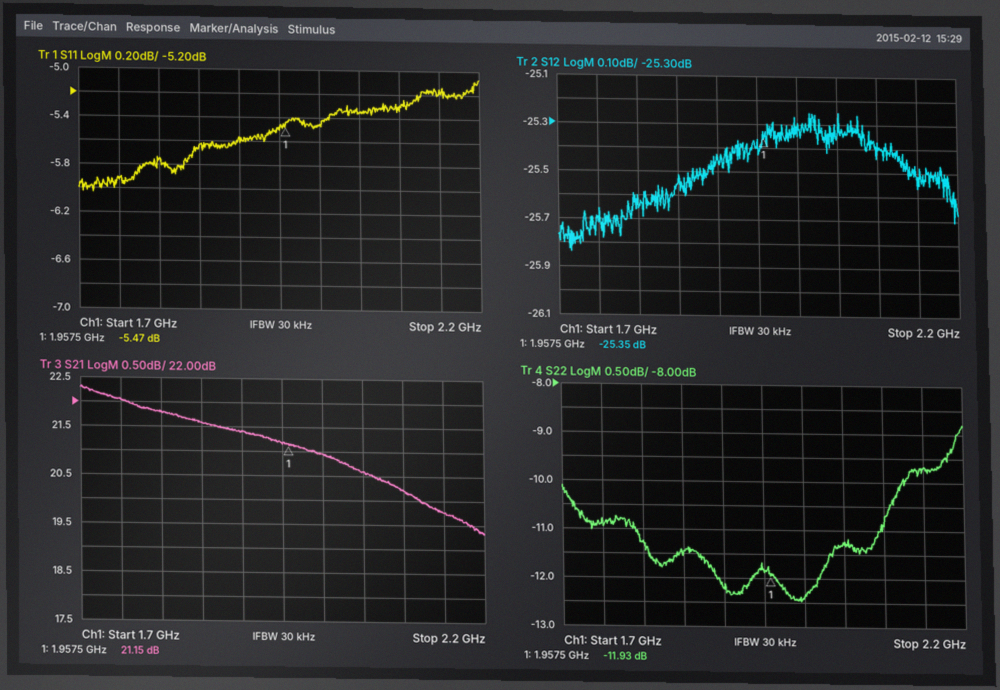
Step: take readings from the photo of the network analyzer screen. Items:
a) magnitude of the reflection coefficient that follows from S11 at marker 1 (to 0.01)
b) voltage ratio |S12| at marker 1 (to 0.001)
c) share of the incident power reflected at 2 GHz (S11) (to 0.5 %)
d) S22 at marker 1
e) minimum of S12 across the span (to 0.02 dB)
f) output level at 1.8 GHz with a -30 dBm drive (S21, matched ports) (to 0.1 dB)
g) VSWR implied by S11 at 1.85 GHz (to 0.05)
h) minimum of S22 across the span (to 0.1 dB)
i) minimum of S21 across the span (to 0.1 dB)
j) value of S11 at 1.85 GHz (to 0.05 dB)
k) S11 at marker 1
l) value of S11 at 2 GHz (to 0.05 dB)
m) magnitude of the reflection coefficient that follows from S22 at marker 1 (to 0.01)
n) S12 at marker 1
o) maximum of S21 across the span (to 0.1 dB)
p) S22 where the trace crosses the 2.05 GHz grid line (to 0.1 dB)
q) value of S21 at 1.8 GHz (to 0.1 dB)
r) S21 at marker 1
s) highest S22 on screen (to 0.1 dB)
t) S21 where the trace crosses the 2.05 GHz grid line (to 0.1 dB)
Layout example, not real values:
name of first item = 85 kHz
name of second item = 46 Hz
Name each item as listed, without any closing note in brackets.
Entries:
magnitude of the reflection coefficient that follows from S11 at marker 1 = 0.53
voltage ratio |S12| at marker 1 = 0.054
share of the incident power reflected at 2 GHz (S11) = 28.5 %
S22 at marker 1 = -11.93 dB
minimum of S12 across the span = -25.84 dB
output level at 1.8 GHz with a -30 dBm drive (S21, matched ports) = -8.2 dBm
VSWR implied by S11 at 1.85 GHz = 3.20
minimum of S22 across the span = -12.5 dB
minimum of S21 across the span = 19.3 dB
value of S11 at 1.85 GHz = -5.65 dB
S11 at marker 1 = -5.47 dB
value of S11 at 2 GHz = -5.45 dB
magnitude of the reflection coefficient that follows from S22 at marker 1 = 0.25
S12 at marker 1 = -25.35 dB
maximum of S21 across the span = 22.3 dB
S22 where the trace crosses the 2.05 GHz grid line = -11.3 dB
value of S21 at 1.8 GHz = 21.8 dB
S21 at marker 1 = 21.15 dB
highest S22 on screen = -8.8 dB
S21 where the trace crosses the 2.05 GHz grid line = 20.6 dB
